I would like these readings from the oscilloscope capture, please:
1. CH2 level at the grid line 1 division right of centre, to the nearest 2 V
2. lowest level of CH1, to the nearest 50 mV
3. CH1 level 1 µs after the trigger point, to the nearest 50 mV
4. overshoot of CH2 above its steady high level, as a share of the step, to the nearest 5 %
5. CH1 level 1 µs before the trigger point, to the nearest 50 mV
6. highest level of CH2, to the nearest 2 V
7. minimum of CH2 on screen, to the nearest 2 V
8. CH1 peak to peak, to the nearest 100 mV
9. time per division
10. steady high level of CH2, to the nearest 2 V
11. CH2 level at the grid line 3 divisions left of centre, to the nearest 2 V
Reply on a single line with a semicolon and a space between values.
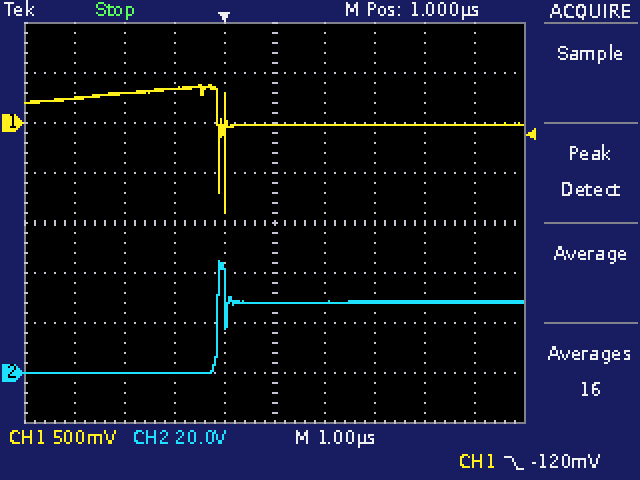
28 V; -900 mV; 0 mV; 60 %; 350 mV; 44 V; 0 V; 1.30 V; 1 µs; 28 V; 0 V
